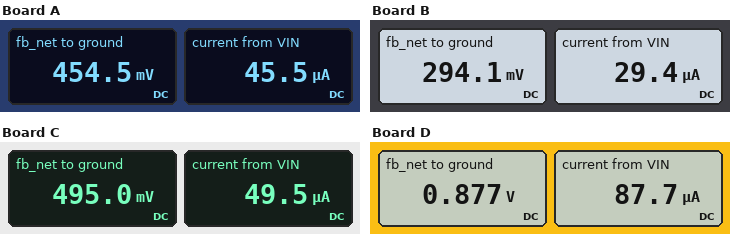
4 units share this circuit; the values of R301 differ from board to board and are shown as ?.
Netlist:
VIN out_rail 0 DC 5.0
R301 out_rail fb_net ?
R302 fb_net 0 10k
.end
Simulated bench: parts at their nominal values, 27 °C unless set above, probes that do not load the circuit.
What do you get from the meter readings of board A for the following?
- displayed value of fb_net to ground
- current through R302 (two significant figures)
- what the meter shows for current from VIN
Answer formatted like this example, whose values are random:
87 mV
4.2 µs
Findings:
454.5 mV
45 µA
45.5 µA
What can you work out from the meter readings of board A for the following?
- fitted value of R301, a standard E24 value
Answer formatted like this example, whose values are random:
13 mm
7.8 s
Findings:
100 kΩ
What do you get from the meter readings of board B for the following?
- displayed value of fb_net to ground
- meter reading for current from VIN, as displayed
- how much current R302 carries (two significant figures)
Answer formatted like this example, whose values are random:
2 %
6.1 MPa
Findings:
294.1 mV
29.4 µA
29 µA
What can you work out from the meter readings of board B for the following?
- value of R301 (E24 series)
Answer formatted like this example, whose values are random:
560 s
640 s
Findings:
160 kΩ
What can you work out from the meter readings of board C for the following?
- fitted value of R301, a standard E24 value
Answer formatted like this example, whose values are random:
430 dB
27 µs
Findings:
91 kΩ
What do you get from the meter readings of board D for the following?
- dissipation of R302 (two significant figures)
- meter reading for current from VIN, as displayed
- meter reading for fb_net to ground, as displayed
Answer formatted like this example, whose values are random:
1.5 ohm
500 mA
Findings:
77 µW
87.7 µA
0.877 V
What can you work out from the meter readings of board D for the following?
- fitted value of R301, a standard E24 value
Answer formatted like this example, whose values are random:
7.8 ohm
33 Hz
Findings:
47 kΩ
